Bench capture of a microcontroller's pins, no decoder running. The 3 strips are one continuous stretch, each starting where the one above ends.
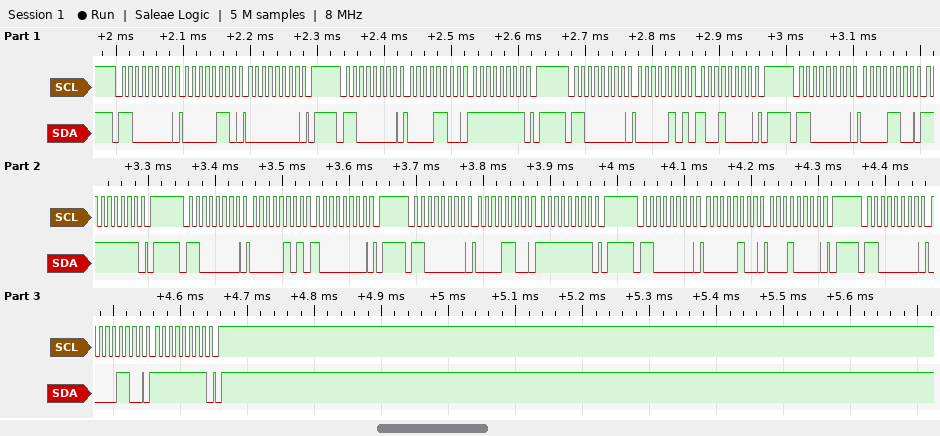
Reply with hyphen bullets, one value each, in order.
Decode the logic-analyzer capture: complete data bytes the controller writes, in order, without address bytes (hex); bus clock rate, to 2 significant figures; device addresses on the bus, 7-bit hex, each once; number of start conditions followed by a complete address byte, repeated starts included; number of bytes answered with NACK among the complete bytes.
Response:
- 06 00 0C FF 05 90 0C FF 05 80 0C FF 04 10 0C FF
- 100 kHz
- 0x60
- 8
- 0
